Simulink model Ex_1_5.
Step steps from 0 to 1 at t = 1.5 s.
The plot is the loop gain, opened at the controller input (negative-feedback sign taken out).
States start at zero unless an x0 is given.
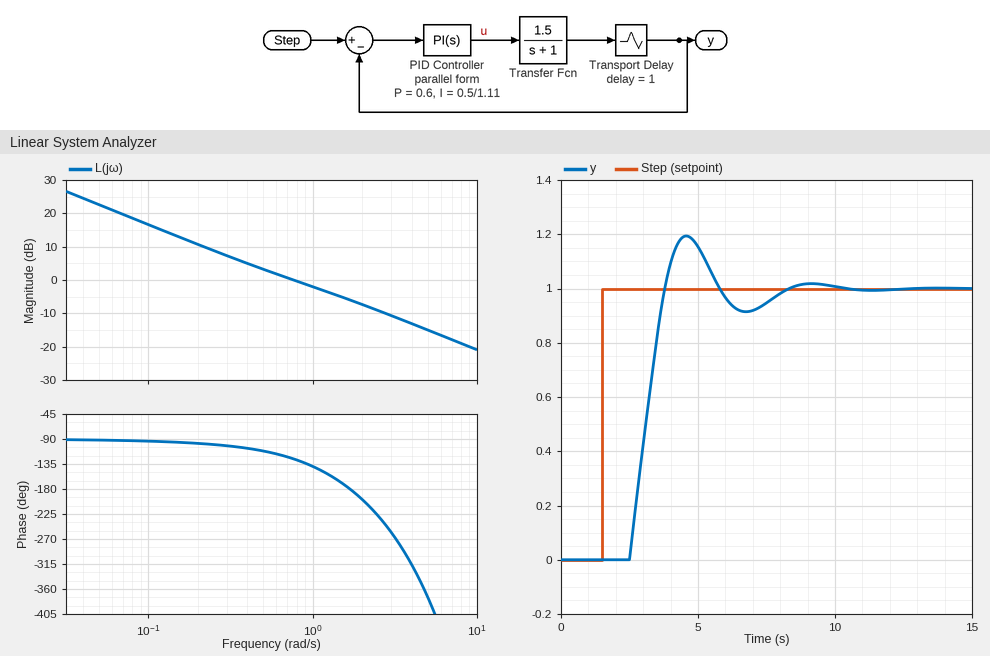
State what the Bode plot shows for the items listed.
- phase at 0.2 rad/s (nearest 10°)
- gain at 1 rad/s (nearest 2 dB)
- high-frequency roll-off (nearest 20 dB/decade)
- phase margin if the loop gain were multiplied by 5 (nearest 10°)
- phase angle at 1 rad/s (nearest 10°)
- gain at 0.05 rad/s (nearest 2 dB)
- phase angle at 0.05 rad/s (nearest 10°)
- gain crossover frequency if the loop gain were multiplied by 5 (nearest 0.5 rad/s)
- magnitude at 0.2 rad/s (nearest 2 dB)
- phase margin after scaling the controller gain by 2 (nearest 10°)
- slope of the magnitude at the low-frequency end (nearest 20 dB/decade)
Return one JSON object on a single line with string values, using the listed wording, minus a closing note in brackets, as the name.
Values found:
{"phase at 0.2 rad/s": "-100°", "gain at 1 rad/s": "-2 dB", "high-frequency roll-off": "-20 dB/decade", "phase margin if the loop gain were multiplied by 5": "-160°", "phase angle at 1 rad/s": "-140°", "gain at 0.05 rad/s": "22 dB", "phase angle at 0.05 rad/s": "-90°", "gain crossover frequency if the loop gain were multiplied by 5": "4.5 rad/s", "magnitude at 0.2 rad/s": "10 dB", "phase margin after scaling the controller gain by 2": "0°", "slope of the magnitude at the low-frequency end": "-20 dB/decade"}
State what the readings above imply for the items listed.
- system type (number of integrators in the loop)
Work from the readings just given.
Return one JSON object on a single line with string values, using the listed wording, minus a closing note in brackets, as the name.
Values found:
{"system type": "1"}
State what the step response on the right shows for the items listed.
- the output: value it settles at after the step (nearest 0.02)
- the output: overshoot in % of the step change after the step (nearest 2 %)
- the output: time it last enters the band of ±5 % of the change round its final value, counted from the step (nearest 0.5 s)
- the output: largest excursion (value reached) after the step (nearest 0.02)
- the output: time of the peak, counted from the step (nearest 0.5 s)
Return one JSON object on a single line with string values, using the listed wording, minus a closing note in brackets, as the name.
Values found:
{"the output: value it settles at after the step": "1.00", "the output: overshoot in % of the step change after the step": "20 %", "the output: time it last enters the band of ±5 % of the change round its final value, counted from the step": "6.0 s", "the output: largest excursion (value reached) after the step": "1.20", "the output: time of the peak, counted from the step": "3.0 s"}
